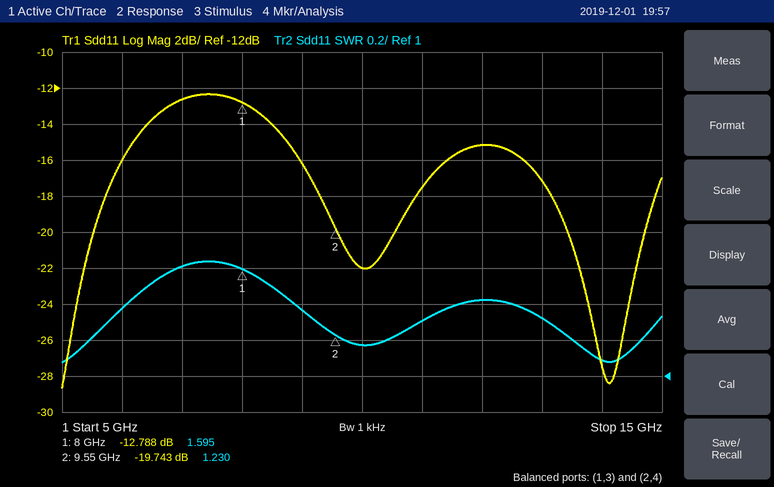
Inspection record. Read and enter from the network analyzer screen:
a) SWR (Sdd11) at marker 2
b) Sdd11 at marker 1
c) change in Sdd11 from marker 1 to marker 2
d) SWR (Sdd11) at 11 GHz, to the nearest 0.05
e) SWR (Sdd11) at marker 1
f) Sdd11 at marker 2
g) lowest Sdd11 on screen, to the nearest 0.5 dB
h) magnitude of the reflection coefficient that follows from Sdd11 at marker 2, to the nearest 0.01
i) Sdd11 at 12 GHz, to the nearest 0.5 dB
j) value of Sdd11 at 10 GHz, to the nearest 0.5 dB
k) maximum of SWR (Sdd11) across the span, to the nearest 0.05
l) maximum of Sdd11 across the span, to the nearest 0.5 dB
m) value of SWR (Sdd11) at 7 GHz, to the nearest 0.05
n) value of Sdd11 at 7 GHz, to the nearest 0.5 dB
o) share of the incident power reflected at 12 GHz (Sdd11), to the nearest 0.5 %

1.230
-12.788 dB
-6.955 dB
1.30
1.595
-19.743 dB
-28.5 dB
0.10
-15.0 dB
-22.0 dB
1.65
-12.5 dB
1.60
-12.5 dB
3.0 %
